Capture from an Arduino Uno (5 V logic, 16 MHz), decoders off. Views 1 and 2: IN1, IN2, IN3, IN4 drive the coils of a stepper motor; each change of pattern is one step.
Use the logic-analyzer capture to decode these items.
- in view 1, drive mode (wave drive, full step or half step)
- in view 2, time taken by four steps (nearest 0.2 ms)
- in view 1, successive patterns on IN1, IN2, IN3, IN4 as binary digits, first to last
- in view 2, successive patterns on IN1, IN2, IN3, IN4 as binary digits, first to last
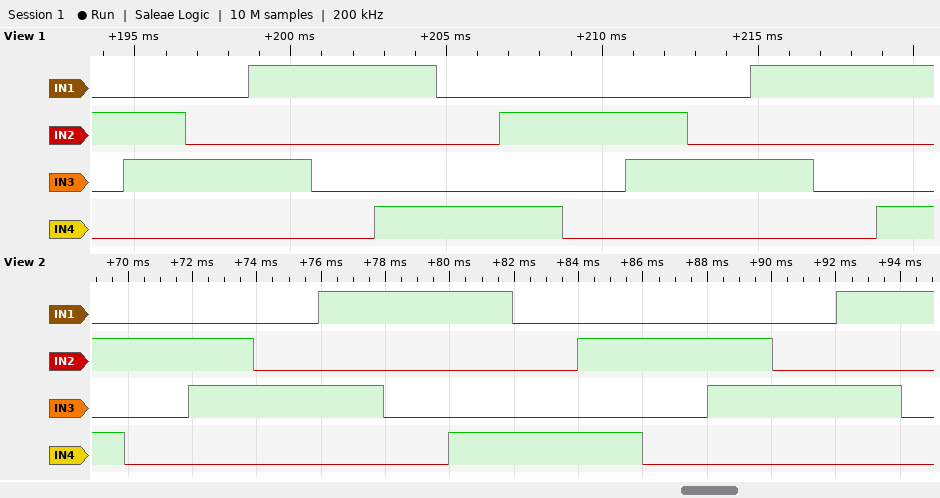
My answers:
half step
8.0 ms
0100 0110 0010 1010 1000 1001 0001 0101 0100 0110 0010 1010 1000 1001
0101 0100 0110 0010 1010 1000 1001 0001 0101 0100 0110 0010 1010 1000
